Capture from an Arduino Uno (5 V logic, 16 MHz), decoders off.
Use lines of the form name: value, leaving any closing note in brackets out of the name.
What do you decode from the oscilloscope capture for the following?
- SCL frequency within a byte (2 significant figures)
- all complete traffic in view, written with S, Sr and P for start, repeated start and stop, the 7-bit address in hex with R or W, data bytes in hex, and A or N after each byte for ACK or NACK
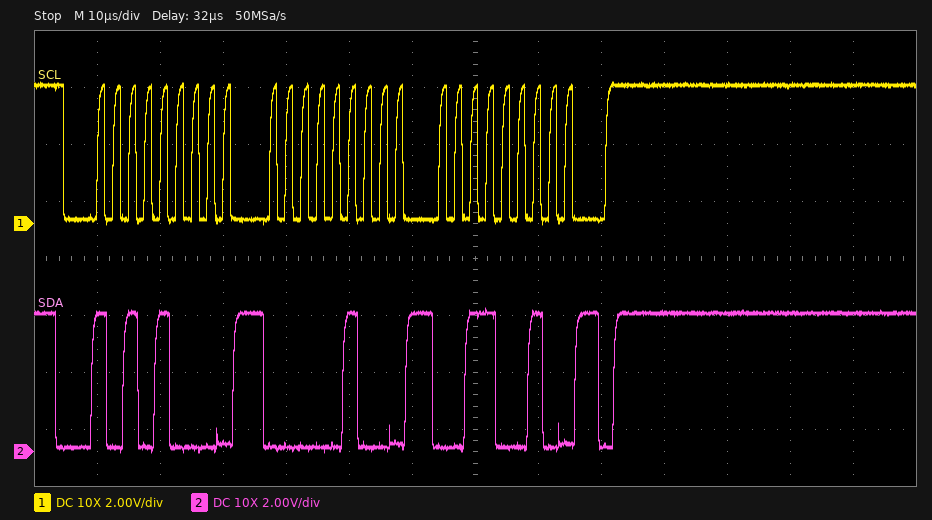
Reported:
SCL frequency within a byte: 400 kHz
all complete traffic in view, written with S, Sr and P for start, repeated start and stop, the 7-bit address in hex with R or W, data bytes in hex, and A or N after each byte for ACK or NACK: S 54W A 04 A 32 A P
